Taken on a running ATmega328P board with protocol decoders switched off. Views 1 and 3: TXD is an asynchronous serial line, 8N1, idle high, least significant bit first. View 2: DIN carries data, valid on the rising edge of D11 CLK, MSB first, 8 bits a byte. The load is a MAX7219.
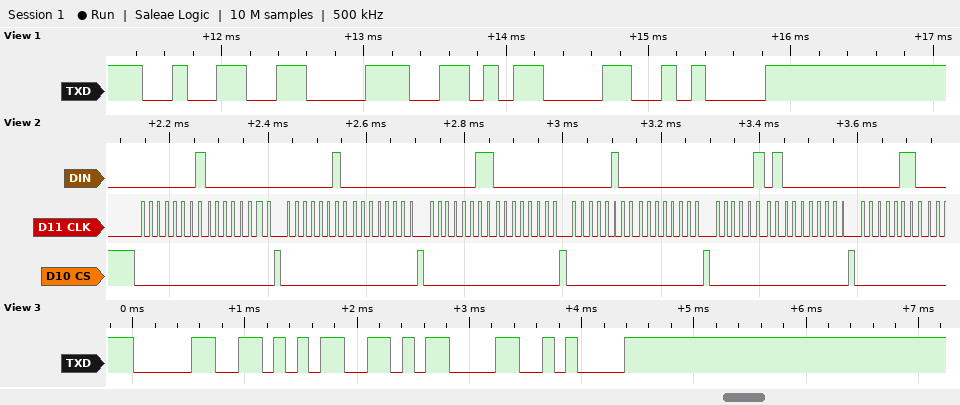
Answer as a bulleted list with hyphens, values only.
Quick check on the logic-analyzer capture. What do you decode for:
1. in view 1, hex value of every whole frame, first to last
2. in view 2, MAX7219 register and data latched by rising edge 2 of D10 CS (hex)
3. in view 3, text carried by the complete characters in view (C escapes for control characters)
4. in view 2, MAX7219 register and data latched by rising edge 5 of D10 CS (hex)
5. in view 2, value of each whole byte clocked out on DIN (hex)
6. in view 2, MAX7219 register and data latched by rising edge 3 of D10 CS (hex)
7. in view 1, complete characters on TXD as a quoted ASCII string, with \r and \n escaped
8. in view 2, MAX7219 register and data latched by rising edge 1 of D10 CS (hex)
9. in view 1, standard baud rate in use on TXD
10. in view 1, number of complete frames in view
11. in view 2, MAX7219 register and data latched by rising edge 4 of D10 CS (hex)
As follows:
- 32 38 0D 0A
- register 0x2, data 0x00
- "05\r\n"
- register 0x5, data 0x00
- 01 00 02 00 03 00 04 00 05 00 06
- register 0x3, data 0x00
- "28\r\n"
- register 0x1, data 0x00
- 9600 baud
- 4
- register 0x4, data 0x00
